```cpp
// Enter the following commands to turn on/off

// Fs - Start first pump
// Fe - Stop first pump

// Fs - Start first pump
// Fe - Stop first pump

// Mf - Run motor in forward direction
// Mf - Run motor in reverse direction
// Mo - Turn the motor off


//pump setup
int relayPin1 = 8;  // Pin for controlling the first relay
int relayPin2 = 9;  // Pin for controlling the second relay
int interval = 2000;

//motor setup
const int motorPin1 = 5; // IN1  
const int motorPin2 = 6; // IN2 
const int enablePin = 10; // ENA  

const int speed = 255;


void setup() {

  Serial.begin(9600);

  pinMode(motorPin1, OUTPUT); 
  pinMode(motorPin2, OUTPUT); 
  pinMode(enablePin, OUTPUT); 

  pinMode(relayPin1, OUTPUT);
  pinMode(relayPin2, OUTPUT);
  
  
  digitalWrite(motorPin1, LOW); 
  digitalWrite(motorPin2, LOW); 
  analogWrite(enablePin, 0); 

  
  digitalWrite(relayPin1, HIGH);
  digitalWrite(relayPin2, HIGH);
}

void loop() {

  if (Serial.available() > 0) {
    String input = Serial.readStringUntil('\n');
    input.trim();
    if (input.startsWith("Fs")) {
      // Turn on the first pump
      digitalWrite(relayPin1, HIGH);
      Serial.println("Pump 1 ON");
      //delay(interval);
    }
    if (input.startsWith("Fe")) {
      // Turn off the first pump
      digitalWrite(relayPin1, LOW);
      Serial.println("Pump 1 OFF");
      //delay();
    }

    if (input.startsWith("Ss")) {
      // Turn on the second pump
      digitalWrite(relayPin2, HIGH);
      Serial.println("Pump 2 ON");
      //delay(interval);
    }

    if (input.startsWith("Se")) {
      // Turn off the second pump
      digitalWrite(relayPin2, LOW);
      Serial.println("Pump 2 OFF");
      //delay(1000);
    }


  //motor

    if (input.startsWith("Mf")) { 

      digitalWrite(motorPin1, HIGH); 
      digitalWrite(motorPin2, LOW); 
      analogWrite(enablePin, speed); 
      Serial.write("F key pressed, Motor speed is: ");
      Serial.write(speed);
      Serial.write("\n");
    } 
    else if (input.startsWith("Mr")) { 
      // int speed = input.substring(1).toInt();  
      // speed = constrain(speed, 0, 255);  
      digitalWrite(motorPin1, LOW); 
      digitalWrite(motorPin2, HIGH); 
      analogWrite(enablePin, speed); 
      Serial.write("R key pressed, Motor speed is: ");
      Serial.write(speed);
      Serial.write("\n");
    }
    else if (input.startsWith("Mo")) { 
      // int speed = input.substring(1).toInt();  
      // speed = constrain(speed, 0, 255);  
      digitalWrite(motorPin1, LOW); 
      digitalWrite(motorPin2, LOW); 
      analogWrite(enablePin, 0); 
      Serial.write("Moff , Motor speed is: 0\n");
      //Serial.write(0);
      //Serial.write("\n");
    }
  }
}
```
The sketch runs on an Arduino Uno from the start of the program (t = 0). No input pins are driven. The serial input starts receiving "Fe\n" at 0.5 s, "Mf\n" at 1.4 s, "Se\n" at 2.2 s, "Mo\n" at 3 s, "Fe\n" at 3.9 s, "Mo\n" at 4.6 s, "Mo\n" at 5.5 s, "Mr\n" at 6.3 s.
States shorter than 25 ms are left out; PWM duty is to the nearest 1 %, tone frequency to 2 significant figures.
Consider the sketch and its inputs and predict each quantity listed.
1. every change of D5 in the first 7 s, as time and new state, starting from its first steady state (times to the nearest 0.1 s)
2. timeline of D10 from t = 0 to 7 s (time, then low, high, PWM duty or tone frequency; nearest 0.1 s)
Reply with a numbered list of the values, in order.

1. 0 s low; 1.4 s high; 3 s low
2. 0 s low; 1.4 s high; 3 s low; 6.3 s high
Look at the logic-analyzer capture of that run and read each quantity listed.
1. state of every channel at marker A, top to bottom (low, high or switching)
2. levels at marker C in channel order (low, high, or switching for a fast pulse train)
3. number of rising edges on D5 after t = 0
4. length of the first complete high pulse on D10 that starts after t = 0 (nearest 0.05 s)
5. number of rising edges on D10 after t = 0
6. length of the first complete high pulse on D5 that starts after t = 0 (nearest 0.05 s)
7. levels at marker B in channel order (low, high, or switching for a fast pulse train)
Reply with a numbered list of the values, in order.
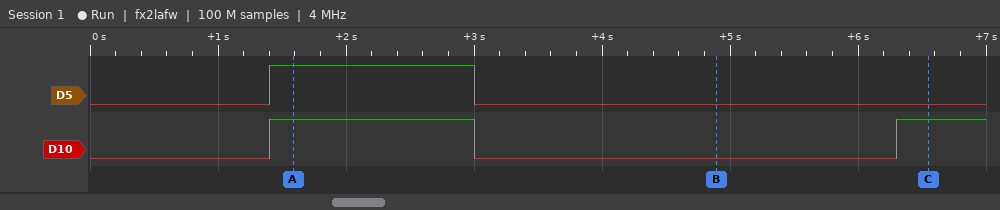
1. D5 high, D10 high
2. D5 low, D10 high
3. 1
4. 1.60 s
5. 2
6. 1.60 s
7. D5 low, D10 low
